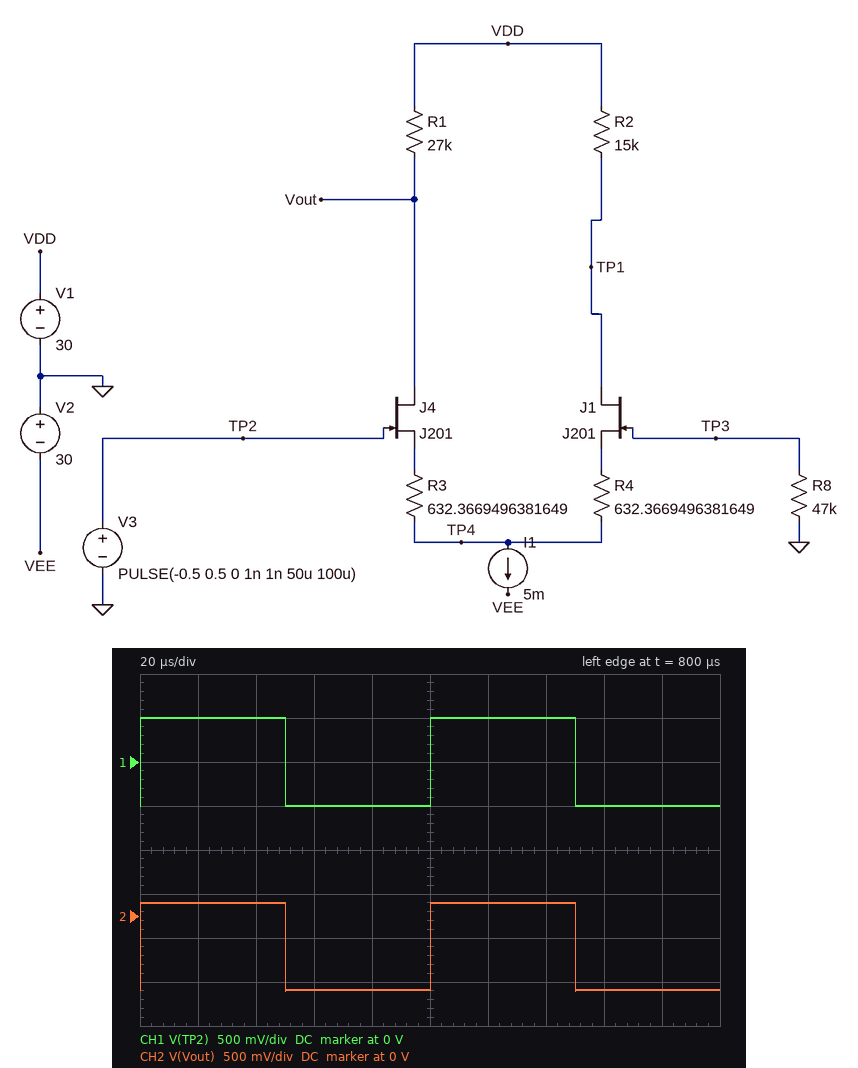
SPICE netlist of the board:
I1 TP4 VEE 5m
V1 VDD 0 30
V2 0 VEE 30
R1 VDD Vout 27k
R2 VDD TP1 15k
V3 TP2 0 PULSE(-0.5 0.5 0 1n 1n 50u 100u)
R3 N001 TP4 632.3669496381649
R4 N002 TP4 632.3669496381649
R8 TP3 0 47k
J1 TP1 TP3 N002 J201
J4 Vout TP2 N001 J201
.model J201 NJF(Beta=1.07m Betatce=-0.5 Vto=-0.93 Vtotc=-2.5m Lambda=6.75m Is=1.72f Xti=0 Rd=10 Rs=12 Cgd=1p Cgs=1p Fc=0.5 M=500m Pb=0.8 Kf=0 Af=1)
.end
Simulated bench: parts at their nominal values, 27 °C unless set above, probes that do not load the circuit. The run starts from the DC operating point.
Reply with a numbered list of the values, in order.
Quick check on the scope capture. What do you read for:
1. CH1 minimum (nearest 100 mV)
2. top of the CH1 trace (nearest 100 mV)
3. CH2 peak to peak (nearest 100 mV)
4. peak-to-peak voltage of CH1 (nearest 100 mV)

1. -500 mV
2. 500 mV
3. 1.0 V
4. 1.0 V
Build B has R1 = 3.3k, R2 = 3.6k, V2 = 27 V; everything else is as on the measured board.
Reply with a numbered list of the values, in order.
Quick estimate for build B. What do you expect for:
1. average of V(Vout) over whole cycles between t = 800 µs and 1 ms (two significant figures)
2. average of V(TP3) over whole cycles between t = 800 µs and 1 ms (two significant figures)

1. 22 V
2. -74 mV
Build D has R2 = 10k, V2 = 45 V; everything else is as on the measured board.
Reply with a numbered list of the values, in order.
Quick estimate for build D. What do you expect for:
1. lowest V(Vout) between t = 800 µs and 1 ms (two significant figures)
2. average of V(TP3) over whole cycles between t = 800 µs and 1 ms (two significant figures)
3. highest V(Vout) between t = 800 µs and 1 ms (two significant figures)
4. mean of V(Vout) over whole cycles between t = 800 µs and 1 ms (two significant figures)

1. -840 mV
2. -280 mV
3. 160 mV
4. -340 mV
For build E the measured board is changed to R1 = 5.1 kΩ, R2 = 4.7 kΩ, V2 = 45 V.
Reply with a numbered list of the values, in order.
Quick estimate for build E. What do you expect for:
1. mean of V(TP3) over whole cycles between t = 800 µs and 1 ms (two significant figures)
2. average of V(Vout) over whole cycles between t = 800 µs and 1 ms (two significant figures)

1. -96 mV
2. 17 V
